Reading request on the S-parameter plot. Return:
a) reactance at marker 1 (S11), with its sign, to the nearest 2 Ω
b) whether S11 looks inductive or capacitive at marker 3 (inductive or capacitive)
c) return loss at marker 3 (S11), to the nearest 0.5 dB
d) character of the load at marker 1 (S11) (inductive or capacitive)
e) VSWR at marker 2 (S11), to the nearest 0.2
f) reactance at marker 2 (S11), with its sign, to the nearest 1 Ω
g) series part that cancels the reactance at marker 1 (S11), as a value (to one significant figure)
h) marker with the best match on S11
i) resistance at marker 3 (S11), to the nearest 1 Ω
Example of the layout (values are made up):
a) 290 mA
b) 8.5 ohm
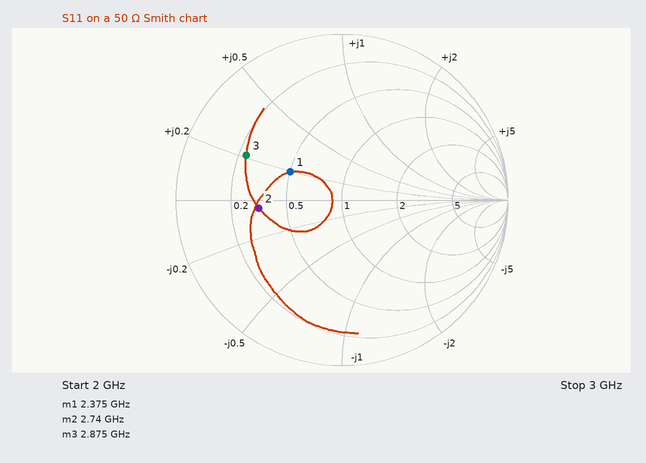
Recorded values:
a) +10 Ω
b) inductive
c) 4.0 dB
d) inductive
e) 3.0
f) -2 Ω
g) 7 pF
h) marker 1
i) 12 Ω
